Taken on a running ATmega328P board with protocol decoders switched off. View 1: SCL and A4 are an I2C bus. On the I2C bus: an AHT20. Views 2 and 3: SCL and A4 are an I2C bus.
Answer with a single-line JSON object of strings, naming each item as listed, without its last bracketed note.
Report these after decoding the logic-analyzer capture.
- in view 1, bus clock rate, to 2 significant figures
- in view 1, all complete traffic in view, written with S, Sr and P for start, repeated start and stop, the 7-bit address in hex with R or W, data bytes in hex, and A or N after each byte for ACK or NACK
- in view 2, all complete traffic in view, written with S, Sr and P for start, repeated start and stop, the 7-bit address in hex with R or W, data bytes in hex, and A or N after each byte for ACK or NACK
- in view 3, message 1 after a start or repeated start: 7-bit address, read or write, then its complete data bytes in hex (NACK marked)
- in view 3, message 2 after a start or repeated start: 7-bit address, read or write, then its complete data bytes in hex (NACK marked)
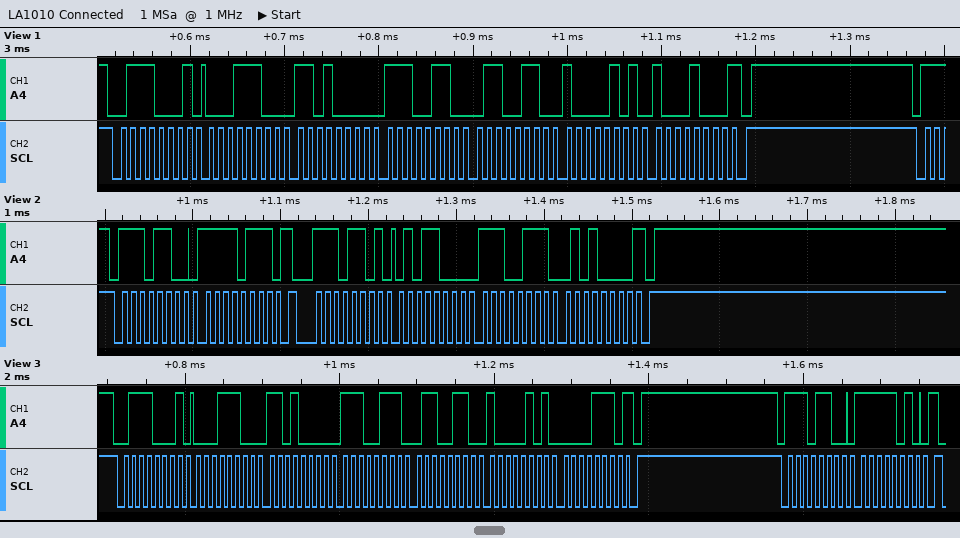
{"in view 1, bus clock rate, to 2 significant figures": "100 kHz", "in view 1, all complete traffic in view, written with S, Sr and P for start, repeated start and stop, the 7-bit address in hex with R or W, data bytes in hex, and A or N after each byte for ACK or NACK": "S 38R A 1C A D0 A E6 A 66 A 85 A 88 N P", "in view 2, all complete traffic in view, written with S, Sr and P for start, repeated start and stop, the 7-bit address in hex with R or W, data bytes in hex, and A or N after each byte for ACK or NACK": "S 76W A F7 A Sr 76R A 58 A E7 A 50 N P", "in view 3, message 1 after a start or repeated start: 7-bit address, read or write, then its complete data bytes in hex": "0x38 read: 1C D0 E7 66 85 0E NACK", "in view 3, message 2 after a start or repeated start: 7-bit address, read or write, then its complete data bytes in hex": "0x76 write: FA"}
